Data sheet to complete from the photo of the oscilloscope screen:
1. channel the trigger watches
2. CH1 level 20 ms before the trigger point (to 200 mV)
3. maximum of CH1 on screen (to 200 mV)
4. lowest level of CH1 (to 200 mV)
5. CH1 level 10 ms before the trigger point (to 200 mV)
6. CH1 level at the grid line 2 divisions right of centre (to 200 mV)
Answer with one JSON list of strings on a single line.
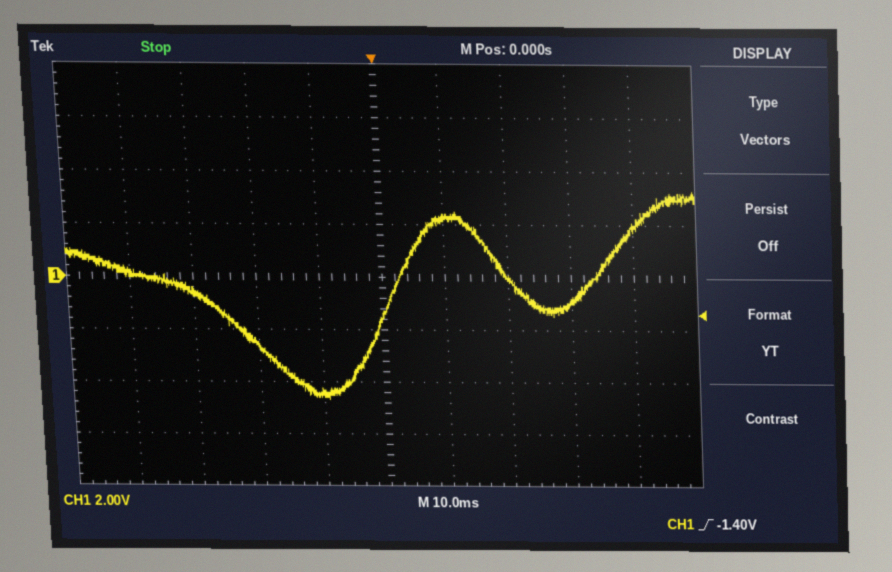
["CH1", "-2.6 V", "3.2 V", "-4.6 V", "-4.4 V", "0.0 V"]
